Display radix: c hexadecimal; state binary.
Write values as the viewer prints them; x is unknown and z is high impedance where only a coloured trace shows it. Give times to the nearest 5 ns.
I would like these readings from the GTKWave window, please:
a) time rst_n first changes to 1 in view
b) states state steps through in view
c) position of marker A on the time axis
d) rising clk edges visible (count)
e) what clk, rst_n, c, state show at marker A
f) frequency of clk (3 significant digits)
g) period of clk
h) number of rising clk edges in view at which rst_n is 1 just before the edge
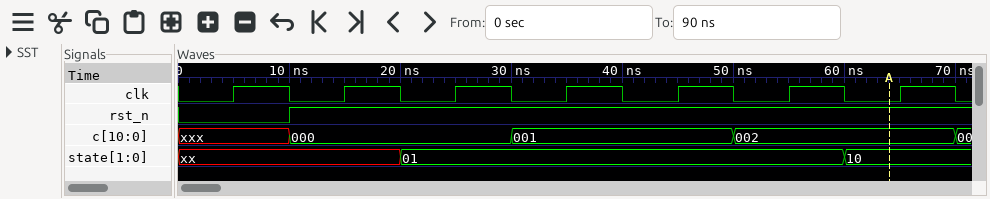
10 ns
xx, 01, 10
65 ns
7
clk=0, rst_n=1, c=002, state=10
100 MHz
10 ns
6
